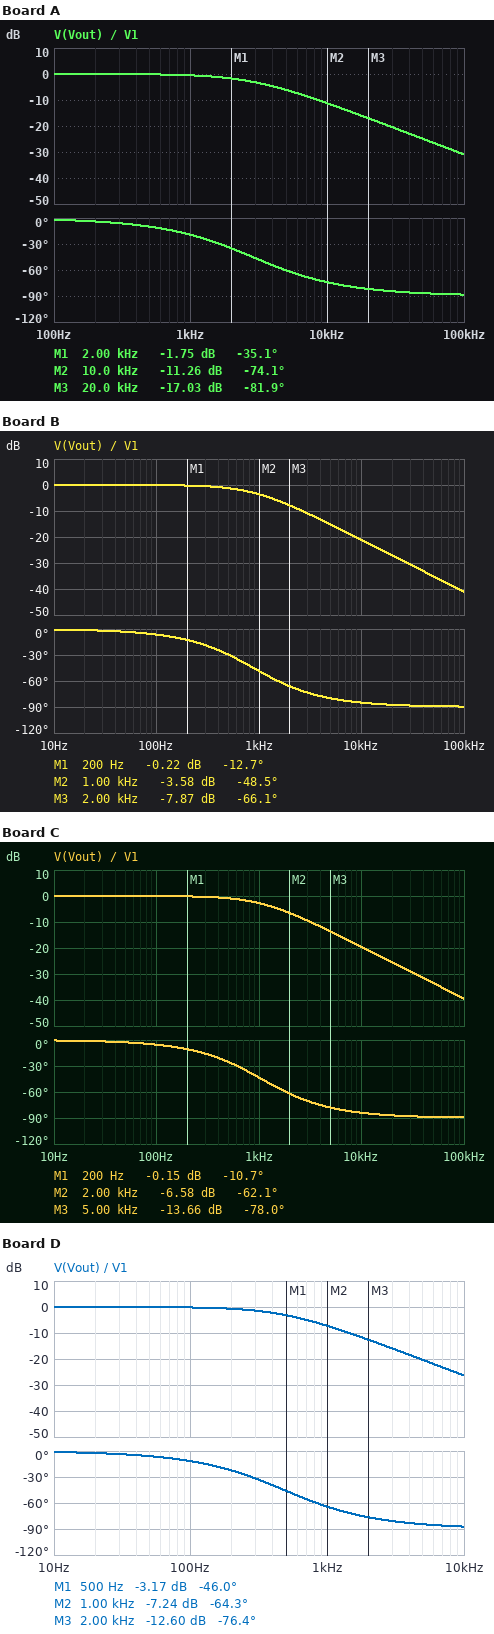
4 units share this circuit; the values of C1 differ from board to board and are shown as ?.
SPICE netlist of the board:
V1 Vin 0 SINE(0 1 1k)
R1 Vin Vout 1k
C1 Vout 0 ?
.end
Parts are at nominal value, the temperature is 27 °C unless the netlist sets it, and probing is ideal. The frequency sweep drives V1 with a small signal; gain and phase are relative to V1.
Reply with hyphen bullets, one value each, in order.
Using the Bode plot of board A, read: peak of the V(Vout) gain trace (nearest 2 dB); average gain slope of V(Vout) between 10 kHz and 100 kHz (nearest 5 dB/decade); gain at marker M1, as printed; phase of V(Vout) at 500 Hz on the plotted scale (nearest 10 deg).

- 0 dB
- -20 dB/decade
- -1.75 dB
- -10 deg
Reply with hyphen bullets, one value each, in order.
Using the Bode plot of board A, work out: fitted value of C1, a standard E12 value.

- 56 nF
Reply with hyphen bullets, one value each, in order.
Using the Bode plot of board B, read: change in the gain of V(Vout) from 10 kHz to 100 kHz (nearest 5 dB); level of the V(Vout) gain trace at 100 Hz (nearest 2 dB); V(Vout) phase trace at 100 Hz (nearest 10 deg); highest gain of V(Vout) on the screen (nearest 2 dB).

- -20 dB
- 0 dB
- -10 deg
- 0 dB
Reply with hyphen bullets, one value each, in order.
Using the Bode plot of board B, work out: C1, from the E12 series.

- 180 nF
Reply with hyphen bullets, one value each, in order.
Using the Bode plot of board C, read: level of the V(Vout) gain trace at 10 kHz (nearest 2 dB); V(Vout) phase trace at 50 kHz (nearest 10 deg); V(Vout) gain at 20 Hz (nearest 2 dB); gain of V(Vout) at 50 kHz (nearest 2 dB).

- -20 dB
- -90 deg
- 0 dB
- -34 dB
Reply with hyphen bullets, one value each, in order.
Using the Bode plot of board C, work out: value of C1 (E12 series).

- 150 nF
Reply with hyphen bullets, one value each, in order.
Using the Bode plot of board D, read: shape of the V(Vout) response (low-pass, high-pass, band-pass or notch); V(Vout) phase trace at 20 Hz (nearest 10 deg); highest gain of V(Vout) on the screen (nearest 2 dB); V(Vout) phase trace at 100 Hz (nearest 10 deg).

- low-pass
- 0 deg
- 0 dB
- -10 deg
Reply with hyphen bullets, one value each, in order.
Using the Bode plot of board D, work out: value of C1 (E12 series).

- 330 nF
